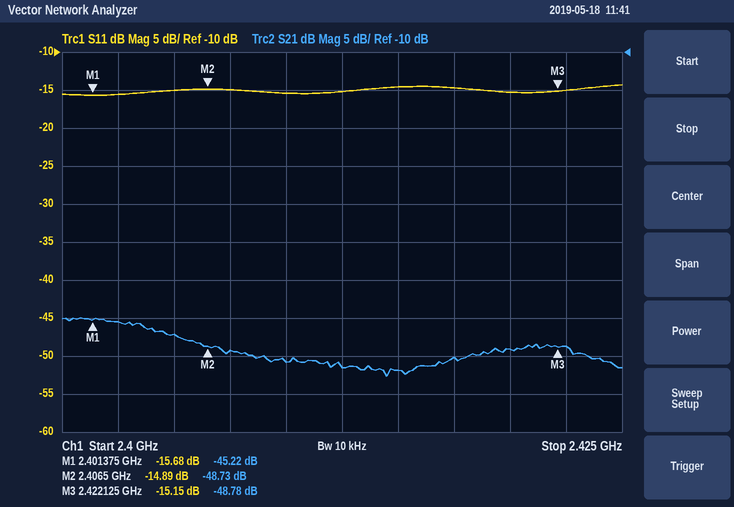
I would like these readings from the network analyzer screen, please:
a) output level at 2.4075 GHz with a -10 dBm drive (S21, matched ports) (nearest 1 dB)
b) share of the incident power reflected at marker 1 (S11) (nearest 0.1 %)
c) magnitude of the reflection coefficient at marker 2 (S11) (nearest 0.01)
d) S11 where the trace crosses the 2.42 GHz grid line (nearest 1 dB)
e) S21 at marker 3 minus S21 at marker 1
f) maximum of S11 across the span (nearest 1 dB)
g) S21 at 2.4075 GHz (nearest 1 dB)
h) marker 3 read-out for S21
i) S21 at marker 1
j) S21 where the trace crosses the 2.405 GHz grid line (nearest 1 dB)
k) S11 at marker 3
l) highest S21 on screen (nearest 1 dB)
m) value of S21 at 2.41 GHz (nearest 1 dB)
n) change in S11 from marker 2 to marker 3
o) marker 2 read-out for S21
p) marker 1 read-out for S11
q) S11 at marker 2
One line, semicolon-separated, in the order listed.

-59 dBm; 2.7 %; 0.18; -15 dB; -3.56 dB; -14 dB; -49 dB; -48.78 dB; -45.22 dB; -47 dB; -15.15 dB; -45 dB; -51 dB; -0.26 dB; -48.73 dB; -15.68 dB; -14.89 dB
